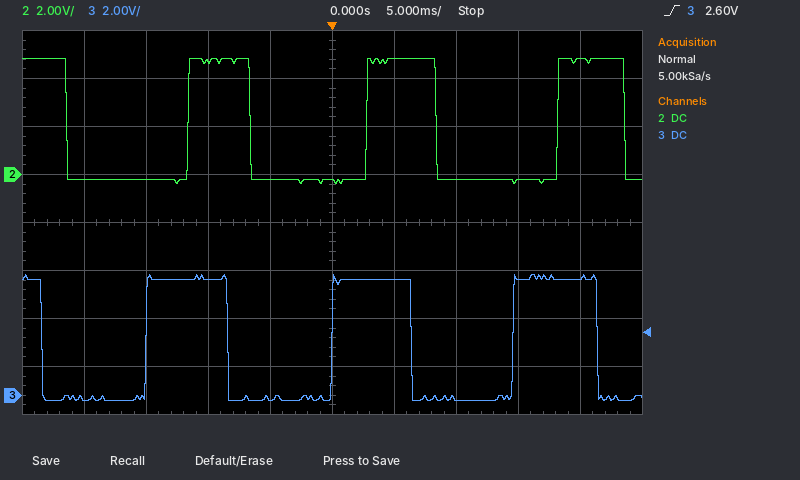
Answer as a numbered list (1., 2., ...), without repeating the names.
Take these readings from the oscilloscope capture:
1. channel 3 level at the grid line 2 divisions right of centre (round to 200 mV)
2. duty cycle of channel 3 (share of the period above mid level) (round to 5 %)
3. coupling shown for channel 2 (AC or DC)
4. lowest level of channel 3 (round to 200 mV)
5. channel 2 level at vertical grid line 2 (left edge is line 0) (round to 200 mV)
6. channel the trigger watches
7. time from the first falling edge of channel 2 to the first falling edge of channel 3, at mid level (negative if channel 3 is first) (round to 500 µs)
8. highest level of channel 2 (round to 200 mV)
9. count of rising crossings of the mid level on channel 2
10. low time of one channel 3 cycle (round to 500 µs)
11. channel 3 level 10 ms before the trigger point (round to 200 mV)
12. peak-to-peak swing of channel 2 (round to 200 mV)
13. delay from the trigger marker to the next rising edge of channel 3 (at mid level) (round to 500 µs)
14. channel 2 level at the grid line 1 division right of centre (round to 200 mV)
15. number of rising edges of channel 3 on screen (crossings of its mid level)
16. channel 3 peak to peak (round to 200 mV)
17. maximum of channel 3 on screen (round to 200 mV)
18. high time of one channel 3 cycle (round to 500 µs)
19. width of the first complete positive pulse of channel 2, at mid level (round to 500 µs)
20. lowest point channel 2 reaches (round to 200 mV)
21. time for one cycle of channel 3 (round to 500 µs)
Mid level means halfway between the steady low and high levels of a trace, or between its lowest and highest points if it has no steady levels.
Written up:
1. -200 mV
2. 45 %
3. DC
4. -200 mV
5. -200 mV
6. channel 3
7. -2.0 ms
8. 4.8 V
9. 3
10. 8.5 ms
11. 4.8 V
12. 5.2 V
13. 14.5 ms
14. 4.8 V
15. 3
16. 5.2 V
17. 5.0 V
18. 6.5 ms
19. 5.0 ms
20. -400 mV
21. 15.0 ms
